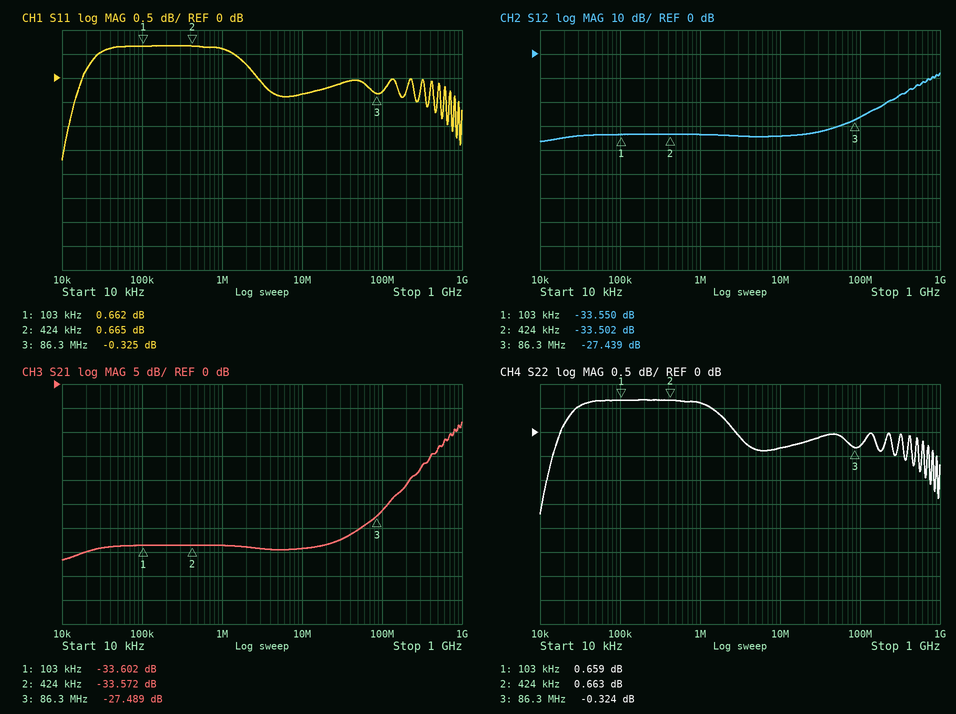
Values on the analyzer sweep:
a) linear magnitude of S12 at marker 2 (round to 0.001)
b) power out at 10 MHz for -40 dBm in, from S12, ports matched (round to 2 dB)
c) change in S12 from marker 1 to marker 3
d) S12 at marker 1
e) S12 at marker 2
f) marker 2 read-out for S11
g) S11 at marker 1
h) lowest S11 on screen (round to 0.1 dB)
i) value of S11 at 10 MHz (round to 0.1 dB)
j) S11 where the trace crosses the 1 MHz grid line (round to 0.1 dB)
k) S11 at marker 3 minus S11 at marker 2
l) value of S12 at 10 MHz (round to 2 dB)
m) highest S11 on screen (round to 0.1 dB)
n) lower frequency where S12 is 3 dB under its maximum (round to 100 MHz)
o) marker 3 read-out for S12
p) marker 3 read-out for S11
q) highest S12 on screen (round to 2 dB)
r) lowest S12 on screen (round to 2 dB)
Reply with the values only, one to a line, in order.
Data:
0.021
-74 dBm
6.111 dB
-33.550 dB
-33.502 dB
0.665 dB
0.662 dB
-1.7 dB
-0.3 dB
0.6 dB
-0.990 dB
-34 dB
0.7 dB
700 MHz
-27.439 dB
-0.325 dB
-8 dB
-36 dB
